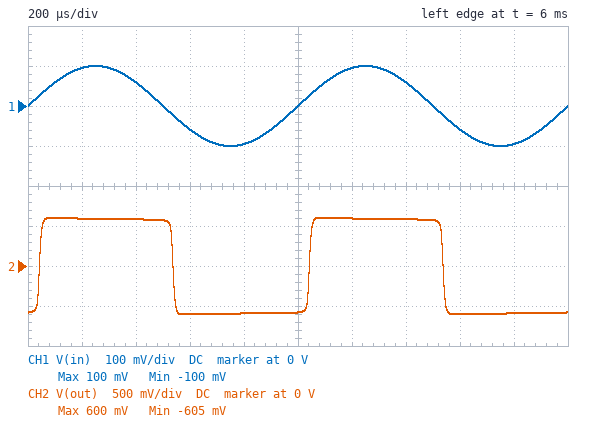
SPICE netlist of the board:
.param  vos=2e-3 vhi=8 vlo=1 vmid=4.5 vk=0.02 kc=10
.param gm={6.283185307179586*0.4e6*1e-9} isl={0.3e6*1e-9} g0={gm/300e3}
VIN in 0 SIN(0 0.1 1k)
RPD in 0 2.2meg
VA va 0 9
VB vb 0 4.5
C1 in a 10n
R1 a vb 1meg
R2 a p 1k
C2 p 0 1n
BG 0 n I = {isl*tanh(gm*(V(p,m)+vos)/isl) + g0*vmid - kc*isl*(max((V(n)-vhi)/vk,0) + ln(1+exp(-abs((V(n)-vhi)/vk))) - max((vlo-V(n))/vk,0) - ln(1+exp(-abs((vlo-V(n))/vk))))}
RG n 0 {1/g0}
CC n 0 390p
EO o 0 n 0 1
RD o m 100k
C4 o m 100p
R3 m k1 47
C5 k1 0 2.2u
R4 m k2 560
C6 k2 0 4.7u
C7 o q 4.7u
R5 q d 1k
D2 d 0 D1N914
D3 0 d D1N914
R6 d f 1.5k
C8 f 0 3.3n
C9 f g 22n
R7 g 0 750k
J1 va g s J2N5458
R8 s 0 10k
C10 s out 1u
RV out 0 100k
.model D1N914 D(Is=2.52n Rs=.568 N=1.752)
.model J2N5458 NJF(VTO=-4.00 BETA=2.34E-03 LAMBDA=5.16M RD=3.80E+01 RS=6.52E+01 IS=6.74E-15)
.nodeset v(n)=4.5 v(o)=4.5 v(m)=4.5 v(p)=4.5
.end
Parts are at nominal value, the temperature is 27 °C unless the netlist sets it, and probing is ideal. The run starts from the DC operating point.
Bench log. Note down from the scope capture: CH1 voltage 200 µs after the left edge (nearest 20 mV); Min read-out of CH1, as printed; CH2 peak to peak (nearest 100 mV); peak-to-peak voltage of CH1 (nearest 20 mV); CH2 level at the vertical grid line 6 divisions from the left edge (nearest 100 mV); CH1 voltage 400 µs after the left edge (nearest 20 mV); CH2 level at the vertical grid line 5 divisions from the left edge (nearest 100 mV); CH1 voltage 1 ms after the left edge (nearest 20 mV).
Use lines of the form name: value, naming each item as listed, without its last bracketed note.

CH1 voltage 200 µs after the left edge: 100 mV
Min read-out of CH1, as printed: -100 mV
CH2 peak to peak: 1.2 V
peak-to-peak voltage of CH1: 200 mV
CH2 level at the vertical grid line 6 divisions from the left edge: 600 mV
CH1 voltage 400 µs after the left edge: 60 mV
CH2 level at the vertical grid line 5 divisions from the left edge: -600 mV
CH1 voltage 1 ms after the left edge: 0 V
